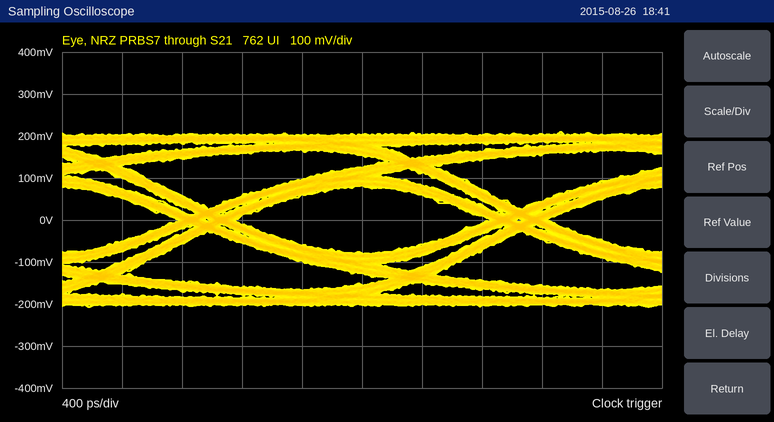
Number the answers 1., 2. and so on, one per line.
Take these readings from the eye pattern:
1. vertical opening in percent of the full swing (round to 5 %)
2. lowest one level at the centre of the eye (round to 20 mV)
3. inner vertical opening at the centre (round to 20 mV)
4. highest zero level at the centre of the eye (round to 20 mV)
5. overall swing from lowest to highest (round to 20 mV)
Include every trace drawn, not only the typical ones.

1. 40 %
2. 80 mV
3. 160 mV
4. -80 mV
5. 420 mV
